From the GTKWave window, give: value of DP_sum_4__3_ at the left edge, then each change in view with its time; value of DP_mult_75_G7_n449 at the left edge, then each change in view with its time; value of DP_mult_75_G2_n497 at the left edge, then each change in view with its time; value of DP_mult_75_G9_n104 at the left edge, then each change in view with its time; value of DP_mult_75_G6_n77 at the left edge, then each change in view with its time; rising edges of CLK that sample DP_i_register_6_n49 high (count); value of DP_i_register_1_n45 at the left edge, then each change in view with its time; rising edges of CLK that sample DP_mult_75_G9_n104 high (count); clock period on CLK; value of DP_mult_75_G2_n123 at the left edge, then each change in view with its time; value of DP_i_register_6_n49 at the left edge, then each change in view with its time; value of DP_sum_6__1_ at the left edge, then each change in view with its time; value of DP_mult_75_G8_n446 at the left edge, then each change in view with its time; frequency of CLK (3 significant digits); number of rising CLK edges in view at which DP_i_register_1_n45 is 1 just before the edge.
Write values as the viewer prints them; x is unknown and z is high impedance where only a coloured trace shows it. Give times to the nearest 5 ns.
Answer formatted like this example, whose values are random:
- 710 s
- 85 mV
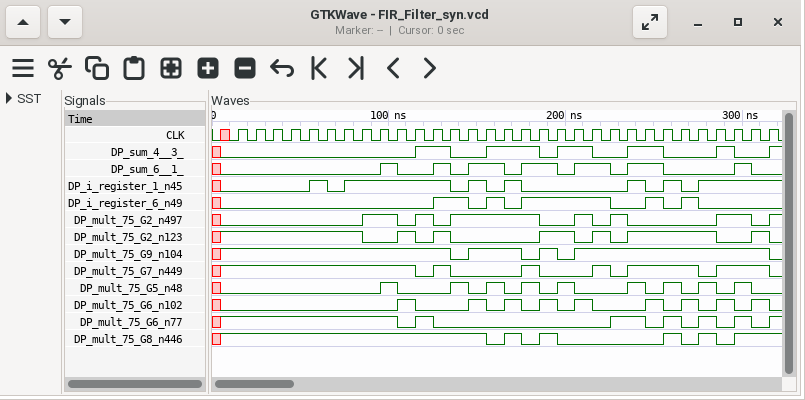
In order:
- x, 0 at 5 ns, 1 at 115 ns, 0 at 135 ns, 1 at 155 ns, 0 at 185 ns, 1 at 195 ns, 0 at 215 ns, 1 at 235 ns, 0 at 255 ns, 1 at 285 ns, 0 at 295 ns, 1 at 315 ns
- x, 1 at 5 ns, 0 at 115 ns, 1 at 125 ns, 0 at 135 ns, 1 at 175 ns, 0 at 185 ns, 1 at 215 ns, 0 at 225 ns, 1 at 235 ns, 0 at 275 ns, 1 at 285 ns, 0 at 315 ns
- x, 0 at 5 ns, 1 at 85 ns, 0 at 105 ns, 1 at 115 ns, 0 at 125 ns, 1 at 135 ns, 0 at 185 ns, 1 at 205 ns, 0 at 215 ns, 1 at 225 ns, 0 at 235 ns, 1 at 285 ns, 0 at 305 ns, 1 at 315 ns
- x, 1 at 5 ns, 0 at 135 ns, 1 at 145 ns, 0 at 175 ns, 1 at 185 ns, 0 at 195 ns, 1 at 205 ns, 0 at 315 ns
- x, 1 at 5 ns, 0 at 105 ns, 1 at 115 ns, 0 at 125 ns, 1 at 225 ns, 0 at 245 ns, 1 at 255 ns, 0 at 265 ns, 1 at 275 ns, 0 at 285 ns, 1 at 295 ns, 0 at 305 ns, 1 at 315 ns
- 10
- x, 0 at 5 ns, 1 at 55 ns, 0 at 65 ns, 1 at 75 ns, 0 at 135 ns, 1 at 145 ns, 0 at 155 ns, 1 at 165 ns, 0 at 175 ns, 1 at 235 ns, 0 at 245 ns, 1 at 255 ns, 0 at 265 ns, 1 at 275 ns
- 28
- 10 ns
- x, 1 at 5 ns, 0 at 85 ns, 1 at 105 ns, 0 at 115 ns, 1 at 125 ns, 0 at 135 ns, 1 at 185 ns, 0 at 205 ns, 1 at 215 ns, 0 at 225 ns, 1 at 235 ns, 0 at 285 ns, 1 at 305 ns, 0 at 315 ns
- x, 0 at 5 ns, 1 at 125 ns, 0 at 145 ns, 1 at 155 ns, 0 at 165 ns, 1 at 175 ns, 0 at 225 ns, 1 at 245 ns, 0 at 255 ns, 1 at 265 ns, 0 at 275 ns
- x, 0 at 5 ns, 1 at 95 ns, 0 at 105 ns, 1 at 125 ns, 0 at 135 ns, 1 at 145 ns, 0 at 165 ns, 1 at 175 ns, 0 at 195 ns, 1 at 205 ns, 0 at 225 ns, 1 at 235 ns, 0 at 255 ns, 1 at 295 ns, 0 at 305 ns
- x, 1 at 5 ns, 0 at 155 ns, 1 at 165 ns, 0 at 175 ns, 1 at 185 ns, 0 at 195 ns, 1 at 255 ns, 0 at 265 ns, 1 at 275 ns, 0 at 285 ns, 1 at 295 ns
- 100 MHz
- 15
